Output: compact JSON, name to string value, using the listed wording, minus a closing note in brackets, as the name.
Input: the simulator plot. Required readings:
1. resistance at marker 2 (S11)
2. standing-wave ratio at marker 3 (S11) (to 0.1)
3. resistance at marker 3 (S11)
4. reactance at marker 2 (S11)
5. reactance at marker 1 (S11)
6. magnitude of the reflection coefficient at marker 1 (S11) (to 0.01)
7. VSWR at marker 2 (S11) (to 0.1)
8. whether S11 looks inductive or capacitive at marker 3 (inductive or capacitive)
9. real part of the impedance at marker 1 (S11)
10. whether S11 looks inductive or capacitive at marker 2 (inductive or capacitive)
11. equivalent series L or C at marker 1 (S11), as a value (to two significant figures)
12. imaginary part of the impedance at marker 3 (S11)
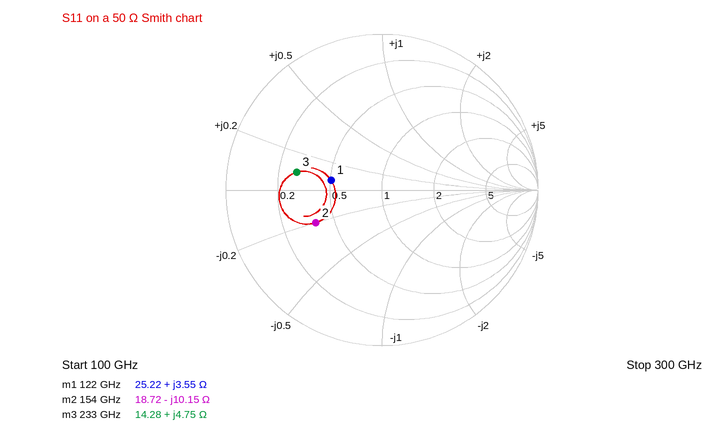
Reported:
{"resistance at marker 2": "18.72 Ω", "standing-wave ratio at marker 3 (S11)": "3.5", "resistance at marker 3": "14.28 Ω", "reactance at marker 2": "-10.15 Ω", "reactance at marker 1": "+3.55 Ω", "magnitude of the reflection coefficient at marker 1 (S11)": "0.33", "VSWR at marker 2 (S11)": "2.8", "whether S11 looks inductive or capacitive at marker 3": "inductive", "real part of the impedance at marker 1": "25.22 Ω", "whether S11 looks inductive or capacitive at marker 2": "capacitive", "equivalent series L or C at marker 1 (S11), as a value": "4.6 pH", "imaginary part of the impedance at marker 3": "+4.75 Ω"}
